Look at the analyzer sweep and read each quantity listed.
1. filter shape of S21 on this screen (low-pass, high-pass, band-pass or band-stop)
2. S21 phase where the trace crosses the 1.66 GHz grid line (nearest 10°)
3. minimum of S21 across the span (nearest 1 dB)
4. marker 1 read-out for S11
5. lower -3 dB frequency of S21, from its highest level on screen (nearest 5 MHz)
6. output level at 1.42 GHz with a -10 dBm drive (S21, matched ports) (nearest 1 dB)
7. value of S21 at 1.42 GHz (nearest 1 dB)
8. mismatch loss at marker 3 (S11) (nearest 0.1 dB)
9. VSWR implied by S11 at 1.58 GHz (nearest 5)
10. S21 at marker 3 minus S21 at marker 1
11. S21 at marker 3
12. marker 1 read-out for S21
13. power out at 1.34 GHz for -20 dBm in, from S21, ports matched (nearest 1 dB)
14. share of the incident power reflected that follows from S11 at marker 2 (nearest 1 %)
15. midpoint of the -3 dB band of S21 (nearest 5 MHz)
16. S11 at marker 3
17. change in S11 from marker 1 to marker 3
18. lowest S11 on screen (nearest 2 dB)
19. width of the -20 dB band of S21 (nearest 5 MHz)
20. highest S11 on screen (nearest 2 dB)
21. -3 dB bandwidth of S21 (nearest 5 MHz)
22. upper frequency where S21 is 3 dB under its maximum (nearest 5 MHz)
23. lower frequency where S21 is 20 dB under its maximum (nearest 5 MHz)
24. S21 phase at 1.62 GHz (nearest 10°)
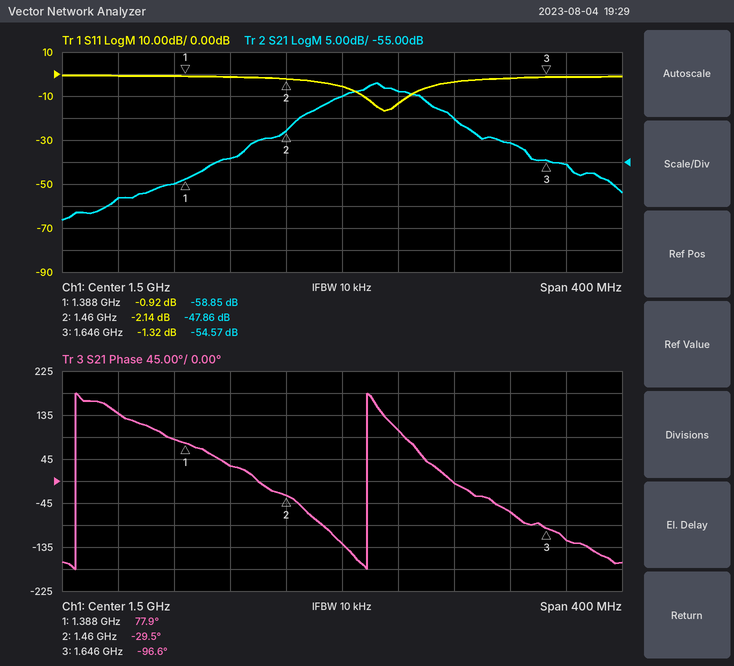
band-pass
-120°
-68 dB
-0.92 dB
1.500 GHz
-64 dBm
-54 dB
5.8 dB
5
4.28 dB
-54.57 dB
-58.85 dB
-83 dBm
61 %
1.530 GHz
-1.32 dB
-0.40 dB
-16 dB
265 MHz
0 dB
55 MHz
1.555 GHz
1.400 GHz
-60°
